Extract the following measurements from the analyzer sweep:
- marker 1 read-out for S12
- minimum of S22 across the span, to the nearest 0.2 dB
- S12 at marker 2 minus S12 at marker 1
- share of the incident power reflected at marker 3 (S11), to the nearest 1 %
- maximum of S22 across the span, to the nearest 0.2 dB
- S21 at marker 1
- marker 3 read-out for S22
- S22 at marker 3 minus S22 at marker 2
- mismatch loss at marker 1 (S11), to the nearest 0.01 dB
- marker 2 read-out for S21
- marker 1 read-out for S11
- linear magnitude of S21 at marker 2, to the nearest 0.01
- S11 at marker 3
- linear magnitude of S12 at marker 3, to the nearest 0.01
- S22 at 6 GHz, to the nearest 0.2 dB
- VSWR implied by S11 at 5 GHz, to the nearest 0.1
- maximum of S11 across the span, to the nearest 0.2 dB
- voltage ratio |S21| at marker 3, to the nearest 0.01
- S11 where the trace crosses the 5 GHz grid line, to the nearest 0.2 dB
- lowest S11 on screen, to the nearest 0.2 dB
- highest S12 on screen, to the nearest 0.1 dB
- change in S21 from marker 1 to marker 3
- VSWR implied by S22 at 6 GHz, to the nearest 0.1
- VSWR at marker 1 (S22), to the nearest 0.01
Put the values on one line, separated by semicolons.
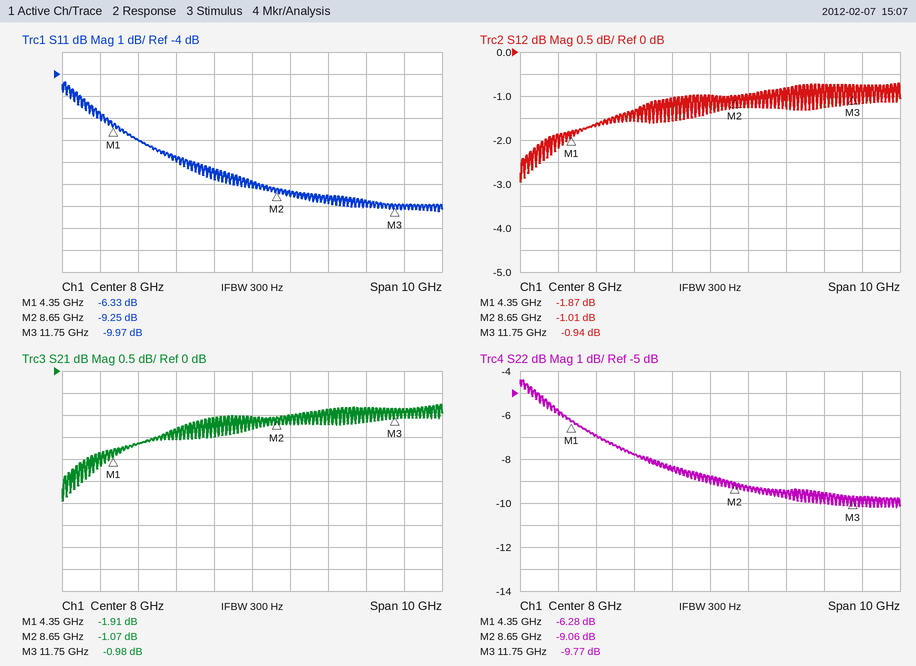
-1.87 dB; -10.2 dB; 0.86 dB; 10 %; -4.4 dB; -1.91 dB; -9.77 dB; -0.71 dB; 1.15 dB; -1.07 dB; -6.33 dB; 0.88; -9.97 dB; 0.90; -7.8 dB; 2.6; -4.4 dB; 0.89; -7.0 dB; -10.2 dB; -0.7 dB; 0.93 dB; 2.4; 2.89
